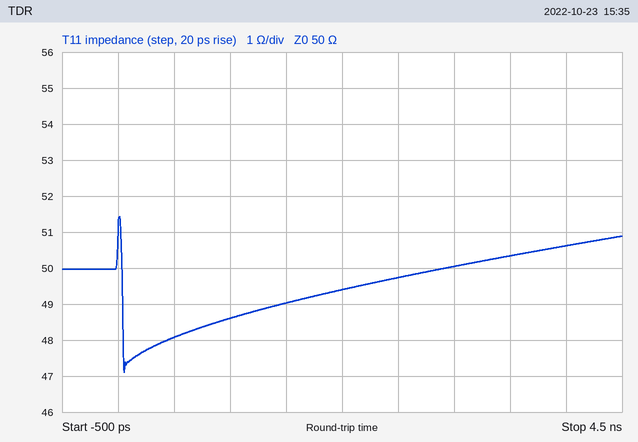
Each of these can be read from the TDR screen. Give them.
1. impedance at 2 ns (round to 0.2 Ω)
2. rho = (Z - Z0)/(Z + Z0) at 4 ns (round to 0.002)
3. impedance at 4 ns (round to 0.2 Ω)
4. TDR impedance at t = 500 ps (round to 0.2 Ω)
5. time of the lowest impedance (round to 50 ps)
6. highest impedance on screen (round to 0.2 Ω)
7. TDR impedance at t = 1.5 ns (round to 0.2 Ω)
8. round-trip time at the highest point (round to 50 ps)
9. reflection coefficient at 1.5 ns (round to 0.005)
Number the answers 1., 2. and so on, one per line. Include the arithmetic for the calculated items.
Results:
1. 49.4 Ω
2. (50.6 − 50)/(50.6 + 50) ≈ +0.006
3. 50.6 Ω
4. 48.0 Ω
5. 50 ps
6. 51.4 Ω
7. 49.0 Ω
8. 0 ps
9. (49 − 50)/(49 + 50) ≈ -0.010
